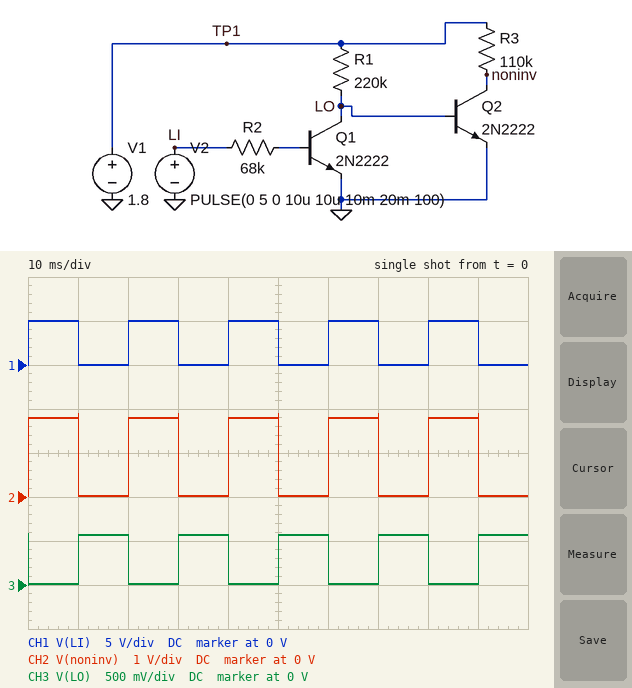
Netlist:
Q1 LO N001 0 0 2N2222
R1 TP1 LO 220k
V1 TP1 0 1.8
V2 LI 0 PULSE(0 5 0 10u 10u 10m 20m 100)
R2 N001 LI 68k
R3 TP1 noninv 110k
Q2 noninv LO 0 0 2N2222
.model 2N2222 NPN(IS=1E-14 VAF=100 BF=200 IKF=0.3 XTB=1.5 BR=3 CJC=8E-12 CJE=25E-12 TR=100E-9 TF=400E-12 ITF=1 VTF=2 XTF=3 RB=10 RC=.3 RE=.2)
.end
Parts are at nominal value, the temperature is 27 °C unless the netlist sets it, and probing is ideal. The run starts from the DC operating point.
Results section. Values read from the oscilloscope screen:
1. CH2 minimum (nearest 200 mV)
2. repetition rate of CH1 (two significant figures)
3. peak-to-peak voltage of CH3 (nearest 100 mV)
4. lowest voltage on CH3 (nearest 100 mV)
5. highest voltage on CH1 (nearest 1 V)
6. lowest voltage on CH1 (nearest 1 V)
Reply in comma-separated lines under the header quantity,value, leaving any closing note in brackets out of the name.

quantity,value
CH2 minimum,0 V
repetition rate of CH1,50 Hz
peak-to-peak voltage of CH3,600 mV
lowest voltage on CH3,0 V
highest voltage on CH1,5 V
lowest voltage on CH1,0 V
